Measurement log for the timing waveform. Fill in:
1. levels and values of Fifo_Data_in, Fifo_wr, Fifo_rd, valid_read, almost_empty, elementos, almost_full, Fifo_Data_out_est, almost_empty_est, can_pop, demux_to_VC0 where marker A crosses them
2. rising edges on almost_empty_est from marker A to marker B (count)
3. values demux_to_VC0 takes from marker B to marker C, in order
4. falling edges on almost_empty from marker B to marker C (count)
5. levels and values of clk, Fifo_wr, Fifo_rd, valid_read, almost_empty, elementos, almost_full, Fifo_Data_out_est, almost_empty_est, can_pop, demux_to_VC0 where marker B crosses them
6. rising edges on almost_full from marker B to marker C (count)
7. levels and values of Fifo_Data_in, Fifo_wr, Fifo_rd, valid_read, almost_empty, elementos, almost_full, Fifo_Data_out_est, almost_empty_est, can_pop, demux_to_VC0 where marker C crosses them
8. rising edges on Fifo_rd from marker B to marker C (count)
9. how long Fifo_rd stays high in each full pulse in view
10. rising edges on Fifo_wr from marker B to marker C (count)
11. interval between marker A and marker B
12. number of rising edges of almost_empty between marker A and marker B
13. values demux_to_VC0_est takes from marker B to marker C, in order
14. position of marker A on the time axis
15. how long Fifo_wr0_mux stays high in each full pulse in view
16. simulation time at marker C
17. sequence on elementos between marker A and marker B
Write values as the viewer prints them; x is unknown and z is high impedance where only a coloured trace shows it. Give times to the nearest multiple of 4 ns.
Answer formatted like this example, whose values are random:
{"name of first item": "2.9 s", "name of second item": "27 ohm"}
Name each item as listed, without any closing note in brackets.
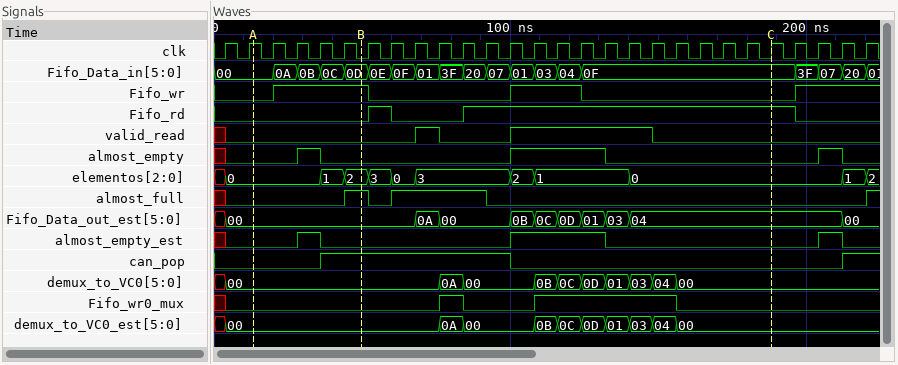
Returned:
{"levels and values of Fifo_Data_in, Fifo_wr, Fifo_rd, valid_read, almost_empty, elementos, almost_full, Fifo_Data_out_est, almost_empty_est, can_pop, demux_to_VC0 where marker A crosses them": "Fifo_Data_in=00, Fifo_wr=0, Fifo_rd=0, valid_read=0, almost_empty=0, elementos=0, almost_full=0, Fifo_Data_out_est=00, almost_empty_est=0, can_pop=0, demux_to_VC0=00", "rising edges on almost_empty_est from marker A to marker B": "1", "values demux_to_VC0 takes from marker B to marker C, in order": "00, 0A, 00, 0B, 0C, 0D, 01, 03, 04, 00", "falling edges on almost_empty from marker B to marker C": "1", "levels and values of clk, Fifo_wr, Fifo_rd, valid_read, almost_empty, elementos, almost_full, Fifo_Data_out_est, almost_empty_est, can_pop, demux_to_VC0 where marker B crosses them": "clk=0, Fifo_wr=1, Fifo_rd=0, valid_read=0, almost_empty=0, elementos=2, almost_full=1, Fifo_Data_out_est=00, almost_empty_est=0, can_pop=1, demux_to_VC0=00", "rising edges on almost_full from marker B to marker C": "1", "levels and values of Fifo_Data_in, Fifo_wr, Fifo_rd, valid_read, almost_empty, elementos, almost_full, Fifo_Data_out_est, almost_empty_est, can_pop, demux_to_VC0 where marker C crosses them": "Fifo_Data_in=0F, Fifo_wr=0, Fifo_rd=1, valid_read=0, almost_empty=0, elementos=0, almost_full=0, Fifo_Data_out_est=04, almost_empty_est=0, can_pop=0, demux_to_VC0=00", "rising edges on Fifo_rd from marker B to marker C": "2", "how long Fifo_rd stays high in each full pulse in view": "8 ns, 112 ns", "rising edges on Fifo_wr from marker B to marker C": "1", "interval between marker A and marker B": "36 ns", "number of rising edges of almost_empty between marker A and marker B": "1", "values demux_to_VC0_est takes from marker B to marker C, in order": "00, 0A, 00, 0B, 0C, 0D, 01, 03, 04, 00", "position of marker A on the time axis": "12 ns", "how long Fifo_wr0_mux stays high in each full pulse in view": "8 ns, 48 ns", "simulation time at marker C": "188 ns", "sequence on elementos between marker A and marker B": "0, 1, 2"}
